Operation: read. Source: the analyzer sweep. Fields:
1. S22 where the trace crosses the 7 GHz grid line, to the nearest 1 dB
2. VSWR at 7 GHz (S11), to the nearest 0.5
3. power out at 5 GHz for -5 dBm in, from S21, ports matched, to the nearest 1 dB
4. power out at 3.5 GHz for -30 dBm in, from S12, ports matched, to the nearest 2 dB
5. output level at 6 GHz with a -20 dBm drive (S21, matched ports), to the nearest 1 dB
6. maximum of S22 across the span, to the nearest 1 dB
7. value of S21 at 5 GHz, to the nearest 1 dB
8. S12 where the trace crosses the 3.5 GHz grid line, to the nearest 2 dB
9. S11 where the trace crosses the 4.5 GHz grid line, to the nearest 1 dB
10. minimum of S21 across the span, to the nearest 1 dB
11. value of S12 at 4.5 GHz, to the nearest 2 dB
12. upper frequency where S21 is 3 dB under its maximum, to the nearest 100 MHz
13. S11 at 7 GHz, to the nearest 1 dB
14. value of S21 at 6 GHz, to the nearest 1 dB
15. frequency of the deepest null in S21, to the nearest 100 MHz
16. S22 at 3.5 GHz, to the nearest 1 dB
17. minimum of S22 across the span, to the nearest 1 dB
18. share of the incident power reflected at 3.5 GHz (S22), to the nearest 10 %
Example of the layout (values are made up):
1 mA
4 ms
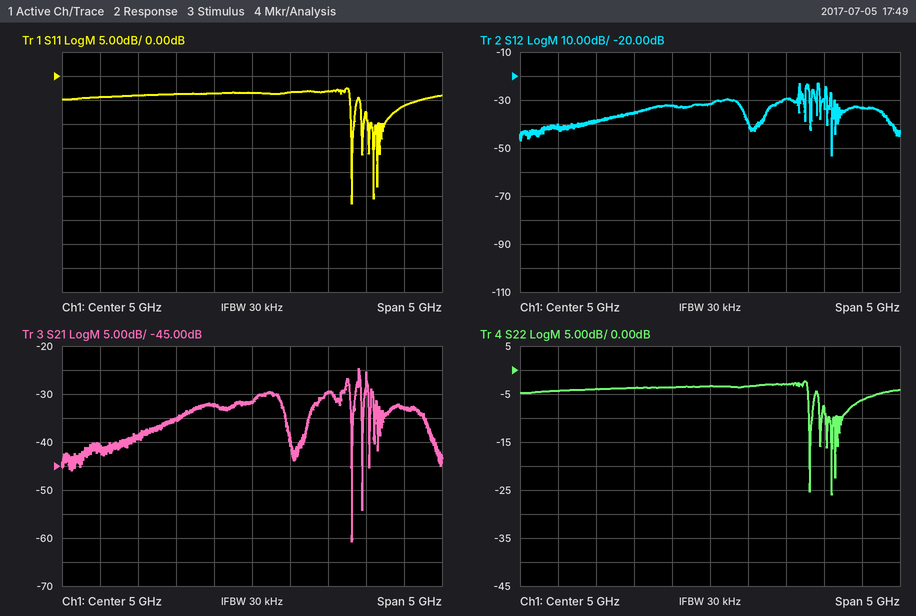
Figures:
-6 dB
3.0
-37 dBm
-68 dBm
-50 dBm
-2 dB
-32 dB
-38 dB
-4 dB
-61 dB
-32 dB
6.4 GHz
-6 dB
-30 dB
6.3 GHz
-4 dB
-26 dB
40 %
